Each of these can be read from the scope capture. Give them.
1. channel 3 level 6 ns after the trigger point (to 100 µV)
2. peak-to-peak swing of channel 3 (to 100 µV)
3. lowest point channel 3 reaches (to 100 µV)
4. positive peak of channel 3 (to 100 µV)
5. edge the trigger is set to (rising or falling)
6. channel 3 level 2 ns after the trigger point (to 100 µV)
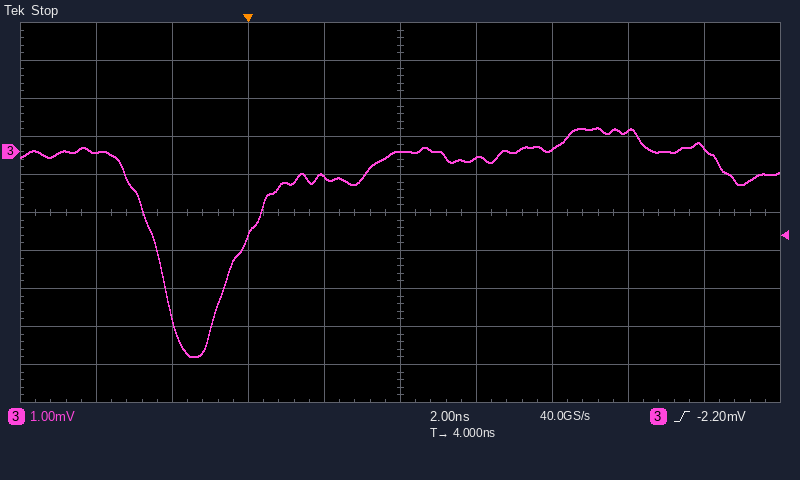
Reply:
-200 µV
6.0 mV
-5.4 mV
600 µV
rising
-700 µV
